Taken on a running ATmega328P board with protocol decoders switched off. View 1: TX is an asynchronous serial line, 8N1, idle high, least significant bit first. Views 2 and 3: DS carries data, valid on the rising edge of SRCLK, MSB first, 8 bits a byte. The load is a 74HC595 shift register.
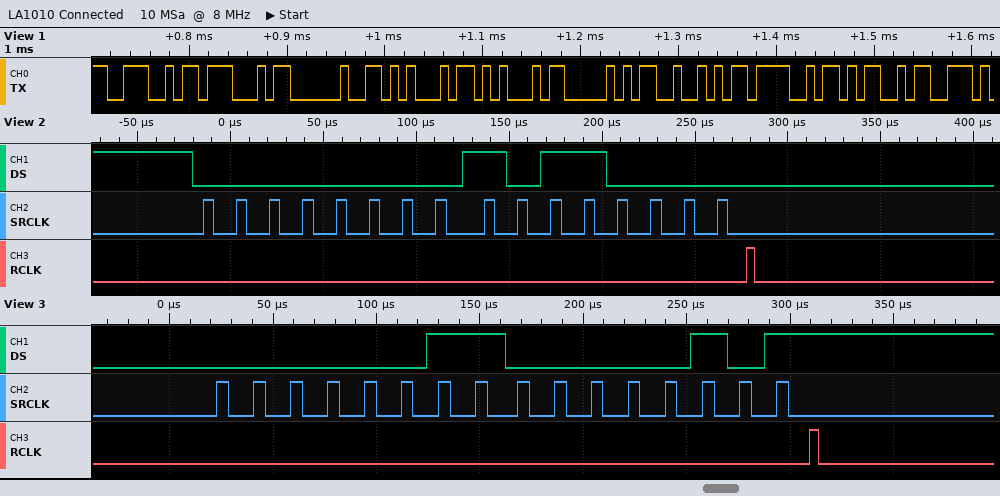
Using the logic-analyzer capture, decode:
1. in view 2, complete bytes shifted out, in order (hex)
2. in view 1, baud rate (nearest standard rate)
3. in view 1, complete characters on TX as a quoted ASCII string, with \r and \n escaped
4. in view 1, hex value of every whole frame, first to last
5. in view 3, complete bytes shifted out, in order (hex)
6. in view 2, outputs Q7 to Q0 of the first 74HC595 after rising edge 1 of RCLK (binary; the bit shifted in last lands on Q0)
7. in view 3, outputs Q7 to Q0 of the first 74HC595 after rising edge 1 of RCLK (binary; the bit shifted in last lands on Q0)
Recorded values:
00 B0
115200 baud
"NG EEPROM"
4E 47 20 45 45 50 52 4F 4D
03 05
10110000
00000101
